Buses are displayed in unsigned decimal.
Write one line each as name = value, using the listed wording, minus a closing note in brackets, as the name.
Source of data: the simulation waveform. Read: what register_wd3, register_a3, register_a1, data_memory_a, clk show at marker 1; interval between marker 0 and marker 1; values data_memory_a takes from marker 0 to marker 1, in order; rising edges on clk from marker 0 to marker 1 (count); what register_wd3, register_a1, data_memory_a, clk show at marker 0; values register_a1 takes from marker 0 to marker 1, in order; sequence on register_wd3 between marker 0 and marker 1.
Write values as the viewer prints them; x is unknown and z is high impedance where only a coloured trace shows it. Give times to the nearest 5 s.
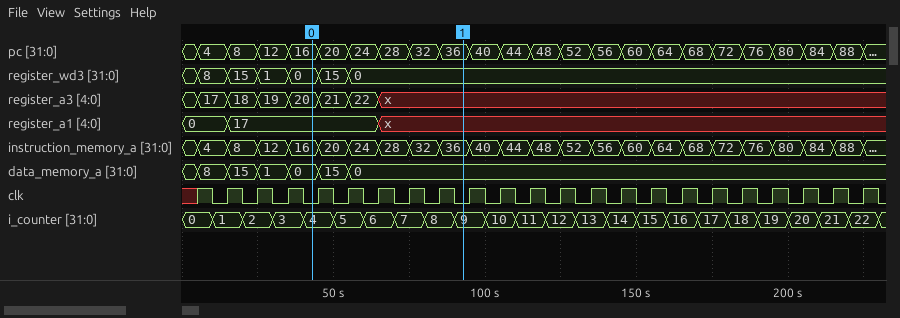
what register_wd3, register_a3, register_a1, data_memory_a, clk show at marker 1 = register_wd3=0, register_a3=x, register_a1=x, data_memory_a=0, clk=0
interval between marker 0 and marker 1 = 50 s
values data_memory_a takes from marker 0 to marker 1, in order = 0, 15, 0
rising edges on clk from marker 0 to marker 1 = 5
what register_wd3, register_a1, data_memory_a, clk show at marker 0 = register_wd3=0, register_a1=17, data_memory_a=0, clk=0
values register_a1 takes from marker 0 to marker 1, in order = 17, x
sequence on register_wd3 between marker 0 and marker 1 = 0, 15, 0
